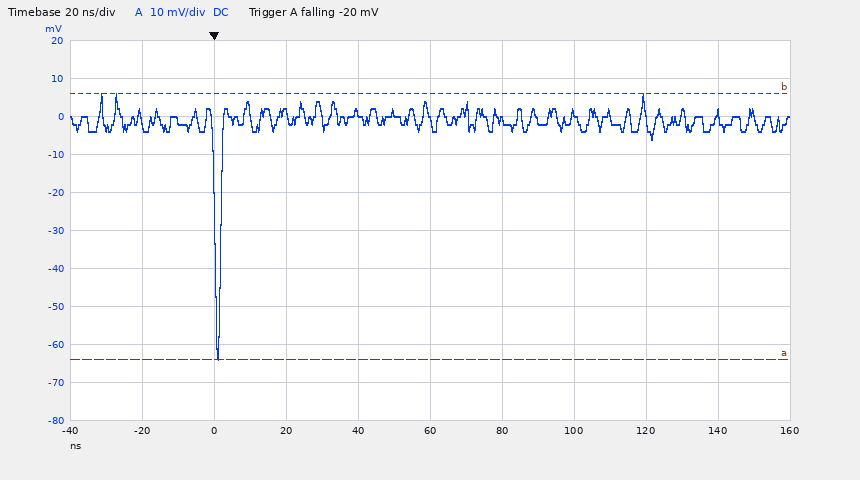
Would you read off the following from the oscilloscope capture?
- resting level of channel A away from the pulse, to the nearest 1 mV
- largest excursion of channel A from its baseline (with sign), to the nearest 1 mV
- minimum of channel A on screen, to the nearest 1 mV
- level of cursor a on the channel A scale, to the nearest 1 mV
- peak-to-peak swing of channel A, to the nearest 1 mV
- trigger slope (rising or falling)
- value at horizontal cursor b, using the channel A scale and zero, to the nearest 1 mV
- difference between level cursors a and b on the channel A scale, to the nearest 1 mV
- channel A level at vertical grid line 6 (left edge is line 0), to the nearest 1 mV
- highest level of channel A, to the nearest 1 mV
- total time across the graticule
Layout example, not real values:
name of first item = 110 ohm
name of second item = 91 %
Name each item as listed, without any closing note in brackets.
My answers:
resting level of channel A away from the pulse, to the nearest 1 mV = -1 mV
largest excursion of channel A from its baseline (with sign), to the nearest 1 mV = -63 mV
minimum of channel A on screen, to the nearest 1 mV = -64 mV
level of cursor a on the channel A scale, to the nearest 1 mV = -64 mV
peak-to-peak swing of channel A, to the nearest 1 mV = 70 mV
trigger slope = falling
value at horizontal cursor b, using the channel A scale and zero, to the nearest 1 mV = 6 mV
difference between level cursors a and b on the channel A scale, to the nearest 1 mV = 70 mV
channel A level at vertical grid line 6 (left edge is line 0), to the nearest 1 mV = -1 mV
highest level of channel A, to the nearest 1 mV = 6 mV
total time across the graticule = 200 ns
